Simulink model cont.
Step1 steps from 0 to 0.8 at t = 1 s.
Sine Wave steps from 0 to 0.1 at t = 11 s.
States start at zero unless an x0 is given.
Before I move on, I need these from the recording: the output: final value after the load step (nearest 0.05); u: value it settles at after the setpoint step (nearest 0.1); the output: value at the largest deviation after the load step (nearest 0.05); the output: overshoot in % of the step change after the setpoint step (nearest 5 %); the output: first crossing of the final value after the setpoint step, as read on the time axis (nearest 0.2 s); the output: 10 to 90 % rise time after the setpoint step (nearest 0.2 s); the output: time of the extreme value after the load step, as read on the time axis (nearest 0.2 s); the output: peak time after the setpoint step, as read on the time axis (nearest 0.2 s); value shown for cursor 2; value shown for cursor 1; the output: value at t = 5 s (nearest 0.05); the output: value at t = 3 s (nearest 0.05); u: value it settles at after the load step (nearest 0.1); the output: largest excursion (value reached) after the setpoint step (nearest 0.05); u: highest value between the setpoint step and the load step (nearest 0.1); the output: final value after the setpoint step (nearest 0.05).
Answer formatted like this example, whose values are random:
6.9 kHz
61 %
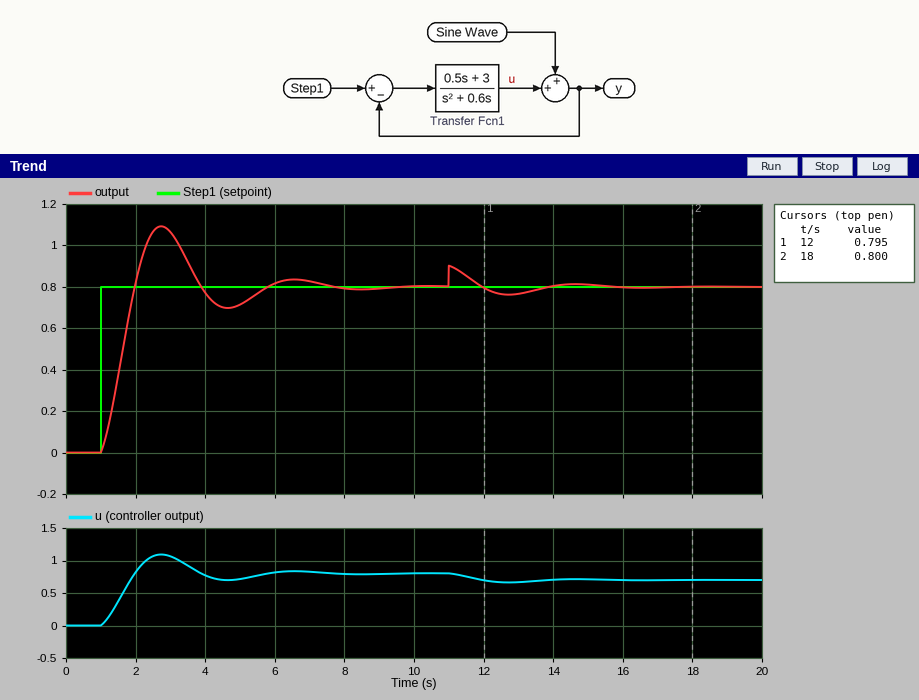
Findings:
0.80
0.8
0.90
35 %
2.0 s
0.8 s
11.0 s
2.8 s
0.800
0.795
0.70
1.05
0.7
1.10
1.1
0.80
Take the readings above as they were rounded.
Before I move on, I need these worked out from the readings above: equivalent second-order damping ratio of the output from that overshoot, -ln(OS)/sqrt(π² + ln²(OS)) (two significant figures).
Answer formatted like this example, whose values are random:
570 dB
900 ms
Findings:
0.32
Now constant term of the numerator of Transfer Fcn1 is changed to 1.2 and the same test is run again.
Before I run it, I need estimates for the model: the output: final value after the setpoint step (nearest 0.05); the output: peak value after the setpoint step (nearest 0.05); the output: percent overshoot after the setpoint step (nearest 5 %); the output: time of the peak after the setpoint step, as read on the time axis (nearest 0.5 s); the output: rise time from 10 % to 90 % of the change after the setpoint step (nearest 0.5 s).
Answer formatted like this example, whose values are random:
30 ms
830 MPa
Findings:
0.80
0.95
20 %
4.0 s
1.5 s
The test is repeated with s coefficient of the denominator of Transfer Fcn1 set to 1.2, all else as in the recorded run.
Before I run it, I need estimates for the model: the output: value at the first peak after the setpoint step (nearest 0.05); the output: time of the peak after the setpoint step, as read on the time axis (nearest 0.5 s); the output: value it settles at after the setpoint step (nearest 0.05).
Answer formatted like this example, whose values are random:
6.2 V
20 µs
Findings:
0.95
3.0 s
0.80
